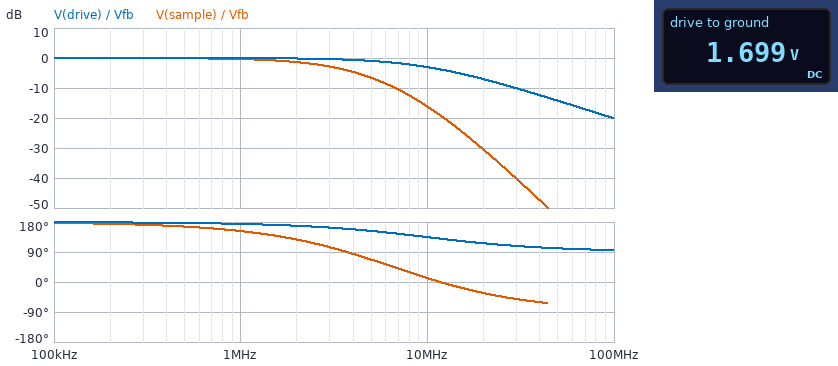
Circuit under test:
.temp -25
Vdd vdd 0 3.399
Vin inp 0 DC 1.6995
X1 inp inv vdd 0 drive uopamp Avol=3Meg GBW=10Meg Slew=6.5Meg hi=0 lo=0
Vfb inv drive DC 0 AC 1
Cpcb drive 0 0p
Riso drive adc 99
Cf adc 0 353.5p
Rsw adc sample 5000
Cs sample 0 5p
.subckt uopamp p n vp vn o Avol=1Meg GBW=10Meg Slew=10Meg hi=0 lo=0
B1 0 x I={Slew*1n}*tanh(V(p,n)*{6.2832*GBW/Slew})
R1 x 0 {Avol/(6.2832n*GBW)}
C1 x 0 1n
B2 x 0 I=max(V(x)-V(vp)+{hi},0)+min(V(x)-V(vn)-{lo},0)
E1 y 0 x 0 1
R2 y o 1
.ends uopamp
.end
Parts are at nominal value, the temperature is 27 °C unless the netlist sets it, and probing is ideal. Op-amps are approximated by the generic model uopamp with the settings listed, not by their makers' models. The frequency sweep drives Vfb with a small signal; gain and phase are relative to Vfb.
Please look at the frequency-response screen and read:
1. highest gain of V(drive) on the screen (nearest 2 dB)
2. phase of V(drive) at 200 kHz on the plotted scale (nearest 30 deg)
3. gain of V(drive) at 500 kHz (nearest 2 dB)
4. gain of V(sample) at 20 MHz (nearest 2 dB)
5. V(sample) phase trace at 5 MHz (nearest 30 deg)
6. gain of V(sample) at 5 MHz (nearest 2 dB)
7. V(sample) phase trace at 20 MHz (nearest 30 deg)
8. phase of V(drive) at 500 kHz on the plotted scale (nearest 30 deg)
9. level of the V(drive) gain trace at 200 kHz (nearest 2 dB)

0 dB
180 deg
0 dB
-30 dB
60 deg
-6 dB
-30 deg
180 deg
0 dB
